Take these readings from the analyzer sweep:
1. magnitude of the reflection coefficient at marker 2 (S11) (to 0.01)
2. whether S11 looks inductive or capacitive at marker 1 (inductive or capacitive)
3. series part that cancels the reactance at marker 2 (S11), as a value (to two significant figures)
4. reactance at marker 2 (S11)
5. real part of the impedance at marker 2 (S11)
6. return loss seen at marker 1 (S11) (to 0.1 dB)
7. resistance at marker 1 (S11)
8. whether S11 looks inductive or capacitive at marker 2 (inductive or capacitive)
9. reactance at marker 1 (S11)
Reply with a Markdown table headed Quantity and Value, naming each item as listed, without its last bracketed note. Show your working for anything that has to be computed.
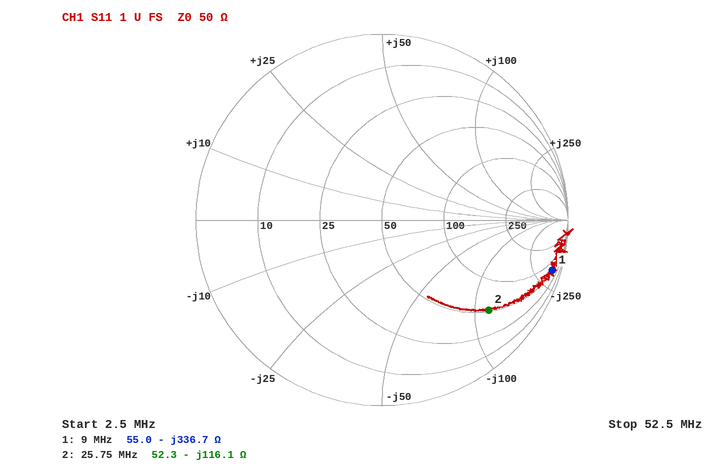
| Quantity | Value |
|---|---|
| magnitude of the reflection coefficient at marker 2 (S11) | 0.75 |
| whether S11 looks inductive or capacitive at marker 1 | capacitive |
| series part that cancels the reactance at marker 2 (S11), as a value | L = 116.1 Ω/(2π × 25.75 MHz) ≈ 718 nH, so 720 nH to two significant figures |
| reactance at marker 2 | -116.1 Ω |
| real part of the impedance at marker 2 | 52.3 Ω |
| return loss seen at marker 1 (S11) | 0.4 dB |
| resistance at marker 1 | 55.0 Ω |
| whether S11 looks inductive or capacitive at marker 2 | capacitive |
| reactance at marker 1 | -336.7 Ω |
